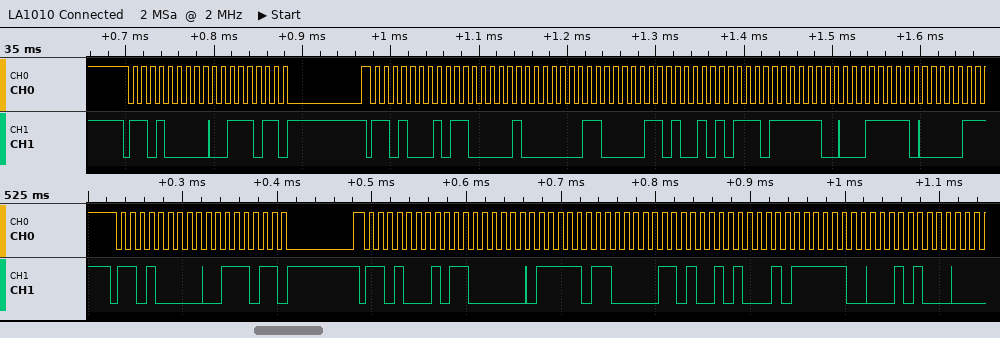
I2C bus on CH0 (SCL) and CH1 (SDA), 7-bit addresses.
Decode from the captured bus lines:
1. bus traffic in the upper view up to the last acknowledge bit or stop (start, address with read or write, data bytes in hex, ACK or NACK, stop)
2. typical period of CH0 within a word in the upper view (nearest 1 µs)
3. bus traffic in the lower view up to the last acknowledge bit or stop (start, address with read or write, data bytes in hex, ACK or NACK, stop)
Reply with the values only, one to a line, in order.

start, address 68 write ACK, 3B ACK, repeated start, address 68 read ACK, C1 ACK, 03 ACK, 0D ACK, 57 ACK, FC ACK, 3E ACK
10 µs
start, address 68 write ACK, 3B ACK, repeated start, address 68 read ACK, C0 ACK, FB ACK, 0D ACK, 51 ACK, FC ACK, 28 ACK
